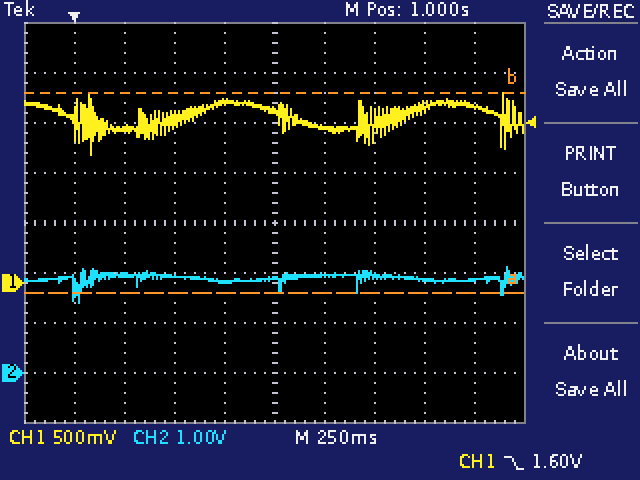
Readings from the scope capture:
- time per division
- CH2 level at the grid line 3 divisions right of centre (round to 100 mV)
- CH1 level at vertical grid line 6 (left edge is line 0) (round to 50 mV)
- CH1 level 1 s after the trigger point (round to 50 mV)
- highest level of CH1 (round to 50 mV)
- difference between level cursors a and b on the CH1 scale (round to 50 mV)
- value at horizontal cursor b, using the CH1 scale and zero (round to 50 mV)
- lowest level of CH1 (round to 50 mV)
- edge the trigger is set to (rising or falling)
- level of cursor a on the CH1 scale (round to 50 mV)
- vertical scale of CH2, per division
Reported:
250 ms
1.9 V
1.55 V
1.70 V
1.90 V
2.00 V
1.90 V
1.30 V
falling
-100 mV
1 V
